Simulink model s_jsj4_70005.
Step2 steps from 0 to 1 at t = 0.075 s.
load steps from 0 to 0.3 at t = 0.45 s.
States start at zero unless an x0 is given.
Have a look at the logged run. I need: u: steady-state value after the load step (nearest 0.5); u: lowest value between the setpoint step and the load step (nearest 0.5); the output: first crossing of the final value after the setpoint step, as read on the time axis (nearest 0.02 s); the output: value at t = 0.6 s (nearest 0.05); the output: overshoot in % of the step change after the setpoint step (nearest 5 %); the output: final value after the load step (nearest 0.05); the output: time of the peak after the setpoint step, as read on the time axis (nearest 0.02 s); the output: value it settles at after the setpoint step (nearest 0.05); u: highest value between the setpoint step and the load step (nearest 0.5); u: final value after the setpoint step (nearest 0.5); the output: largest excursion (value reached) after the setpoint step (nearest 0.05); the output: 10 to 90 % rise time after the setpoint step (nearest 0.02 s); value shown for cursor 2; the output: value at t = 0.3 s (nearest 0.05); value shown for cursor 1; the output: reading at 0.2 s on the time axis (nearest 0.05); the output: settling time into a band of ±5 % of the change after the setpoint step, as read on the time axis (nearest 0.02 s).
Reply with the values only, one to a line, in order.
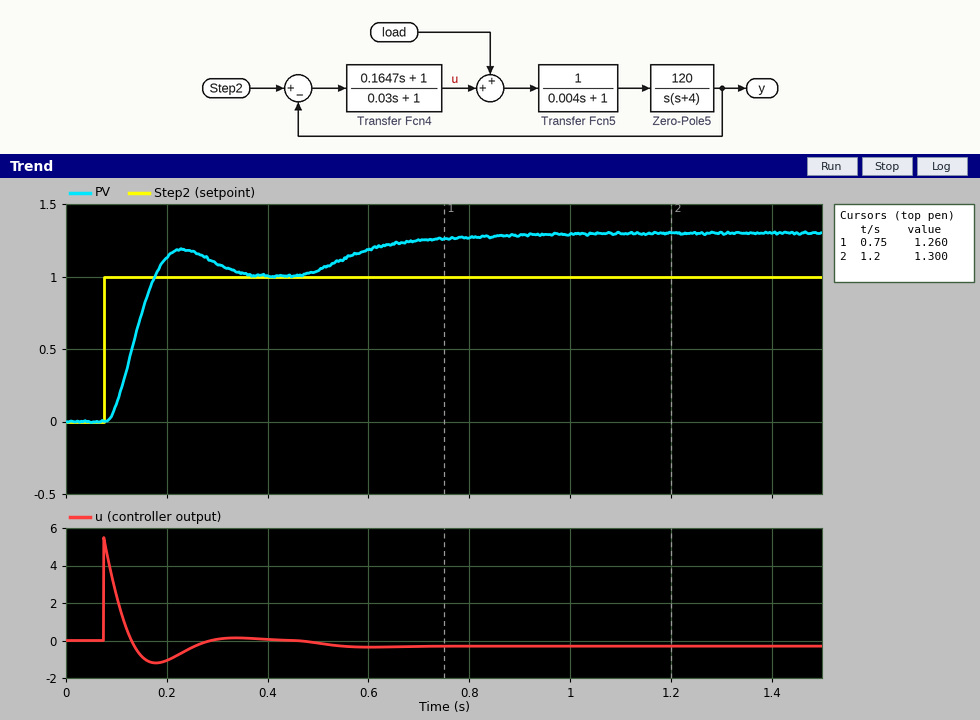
-0.5
-1.0
0.18 s
1.20
20 %
1.30
0.24 s
1.00
5.5
0.0
1.20
0.06 s
1.300
1.10
1.260
1.15
0.32 s
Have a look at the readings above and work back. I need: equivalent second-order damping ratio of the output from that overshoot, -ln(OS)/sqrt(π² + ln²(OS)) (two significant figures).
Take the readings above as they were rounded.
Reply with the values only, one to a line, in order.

0.46
